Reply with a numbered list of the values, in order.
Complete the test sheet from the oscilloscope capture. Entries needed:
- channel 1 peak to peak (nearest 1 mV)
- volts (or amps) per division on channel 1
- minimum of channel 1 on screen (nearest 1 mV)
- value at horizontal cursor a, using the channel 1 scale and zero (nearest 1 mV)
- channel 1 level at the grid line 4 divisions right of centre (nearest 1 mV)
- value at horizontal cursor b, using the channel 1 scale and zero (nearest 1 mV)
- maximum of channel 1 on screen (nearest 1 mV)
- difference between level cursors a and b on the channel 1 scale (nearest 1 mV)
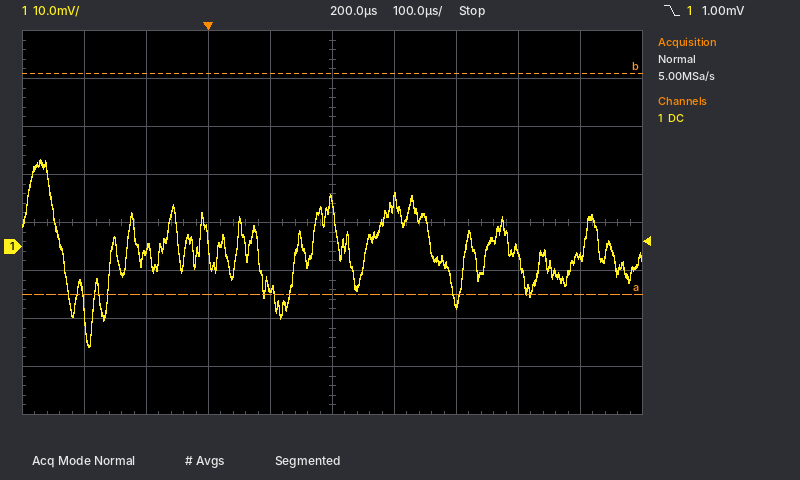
1. 39 mV
2. 10 mV
3. -21 mV
4. -10 mV
5. -2 mV
6. 36 mV
7. 18 mV
8. 46 mV
